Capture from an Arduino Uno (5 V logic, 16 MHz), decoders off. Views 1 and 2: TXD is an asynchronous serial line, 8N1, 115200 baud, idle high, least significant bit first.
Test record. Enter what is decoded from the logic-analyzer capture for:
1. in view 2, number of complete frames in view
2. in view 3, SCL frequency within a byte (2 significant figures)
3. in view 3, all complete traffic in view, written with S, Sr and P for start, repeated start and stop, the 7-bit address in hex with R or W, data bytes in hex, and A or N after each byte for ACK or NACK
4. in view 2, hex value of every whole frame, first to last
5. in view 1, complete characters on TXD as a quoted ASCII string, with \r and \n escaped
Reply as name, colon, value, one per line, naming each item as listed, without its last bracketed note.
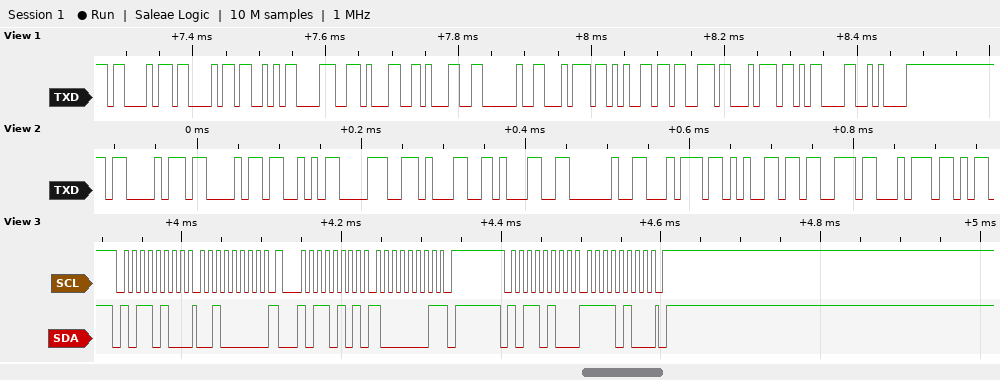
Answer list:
in view 2, number of complete frames in view: 11
in view 3, SCL frequency within a byte: 100 kHz
in view 3, all complete traffic in view, written with S, Sr and P for start, repeated start and stop, the 7-bit address in hex with R or W, data bytes in hex, and A or N after each byte for ACK or NACK: S 5AW A 20 A Sr 5AR A 81 N P S 5AW A F4 A P
in view 2, hex value of every whole frame, first to last: 0x43 0x43 0x53 0x38 0x31 0x31 0x20 0x74 0x65 0x73 0x74
in view 1, complete characters on TXD as a quoted ASCII string, with \r and \n escaped: "CCS811 test\r\n"
